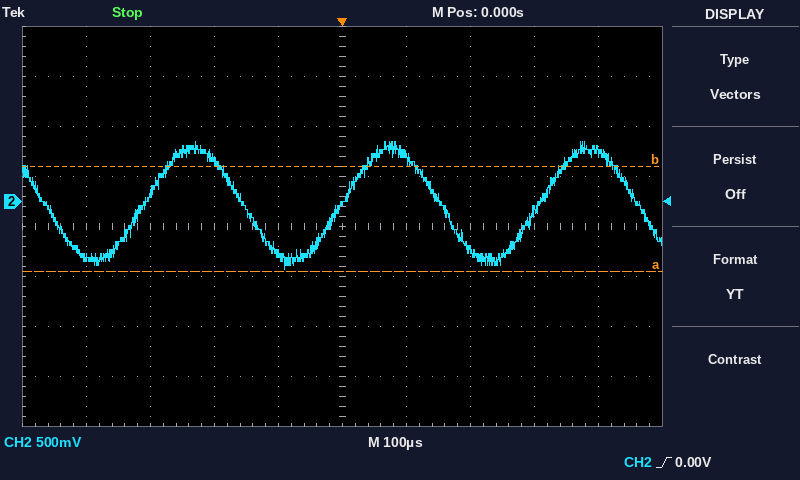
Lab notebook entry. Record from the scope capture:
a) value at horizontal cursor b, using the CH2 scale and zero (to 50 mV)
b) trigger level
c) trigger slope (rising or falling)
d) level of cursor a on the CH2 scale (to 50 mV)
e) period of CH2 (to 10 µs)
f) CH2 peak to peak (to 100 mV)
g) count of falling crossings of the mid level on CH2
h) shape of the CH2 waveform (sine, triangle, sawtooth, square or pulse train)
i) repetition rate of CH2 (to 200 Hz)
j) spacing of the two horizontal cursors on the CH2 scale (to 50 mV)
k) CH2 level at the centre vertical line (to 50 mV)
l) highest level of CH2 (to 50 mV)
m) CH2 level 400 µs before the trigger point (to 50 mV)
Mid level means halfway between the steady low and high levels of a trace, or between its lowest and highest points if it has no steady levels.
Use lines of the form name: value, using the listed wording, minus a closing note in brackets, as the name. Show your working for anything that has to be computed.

value at horizontal cursor b, using the CH2 scale and zero: 350 mV
trigger level: 0.00 V
trigger slope: rising
level of cursor a on the CH2 scale: -700 mV
period of CH2: 310 µs
CH2 peak to peak: 1.30 V
count of falling crossings of the mid level on CH2: 4
shape of the CH2 waveform: sine
repetition rate of CH2: 1 / 310 µs ≈ 3.2 kHz
spacing of the two horizontal cursors on the CH2 scale: 1.05 V
CH2 level at the centre vertical line: -50 mV
highest level of CH2: 600 mV
CH2 level 400 µs before the trigger point: -550 mV
